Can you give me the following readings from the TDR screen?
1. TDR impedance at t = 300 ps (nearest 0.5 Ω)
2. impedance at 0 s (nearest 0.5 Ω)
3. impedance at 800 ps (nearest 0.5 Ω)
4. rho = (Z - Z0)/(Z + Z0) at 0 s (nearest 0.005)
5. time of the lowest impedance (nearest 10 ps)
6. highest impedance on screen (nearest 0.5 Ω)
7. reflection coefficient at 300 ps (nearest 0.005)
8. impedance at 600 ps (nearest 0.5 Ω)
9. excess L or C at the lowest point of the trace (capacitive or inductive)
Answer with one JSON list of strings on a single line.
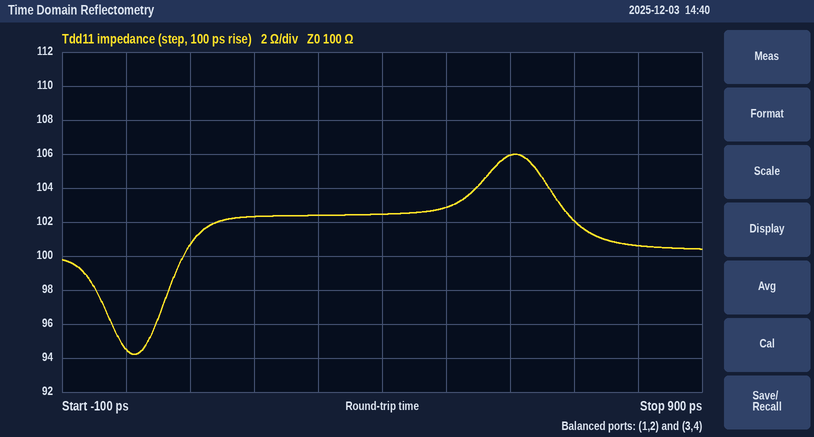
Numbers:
["102.5 Ω", "94.5 Ω", "100.5 Ω", "-0.030", "10 ps", "106.0 Ω", "+0.010", "106.0 Ω", "capacitive"]
